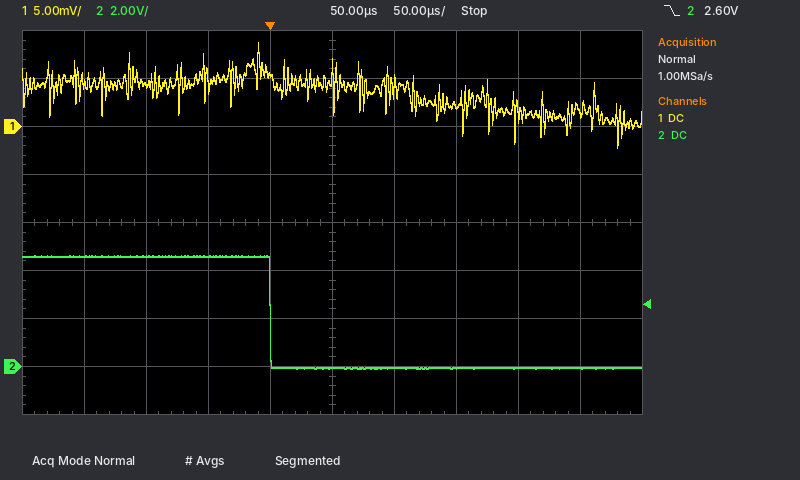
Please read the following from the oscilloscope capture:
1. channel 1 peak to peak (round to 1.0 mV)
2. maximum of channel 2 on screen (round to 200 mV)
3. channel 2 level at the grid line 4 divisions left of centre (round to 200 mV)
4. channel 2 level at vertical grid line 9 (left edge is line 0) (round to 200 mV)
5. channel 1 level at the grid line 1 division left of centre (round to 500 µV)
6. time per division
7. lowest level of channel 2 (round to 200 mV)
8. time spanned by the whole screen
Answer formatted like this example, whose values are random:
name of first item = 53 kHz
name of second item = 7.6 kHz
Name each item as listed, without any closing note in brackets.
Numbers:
channel 1 peak to peak = 11.0 mV
maximum of channel 2 on screen = 4.6 V
channel 2 level at the grid line 4 divisions left of centre = 4.6 V
channel 2 level at vertical grid line 9 (left edge is line 0) = 0.0 V
channel 1 level at the grid line 1 division left of centre = 5.5 mV
time per division = 50 µs
lowest level of channel 2 = 0.0 V
time spanned by the whole screen = 500 µs
